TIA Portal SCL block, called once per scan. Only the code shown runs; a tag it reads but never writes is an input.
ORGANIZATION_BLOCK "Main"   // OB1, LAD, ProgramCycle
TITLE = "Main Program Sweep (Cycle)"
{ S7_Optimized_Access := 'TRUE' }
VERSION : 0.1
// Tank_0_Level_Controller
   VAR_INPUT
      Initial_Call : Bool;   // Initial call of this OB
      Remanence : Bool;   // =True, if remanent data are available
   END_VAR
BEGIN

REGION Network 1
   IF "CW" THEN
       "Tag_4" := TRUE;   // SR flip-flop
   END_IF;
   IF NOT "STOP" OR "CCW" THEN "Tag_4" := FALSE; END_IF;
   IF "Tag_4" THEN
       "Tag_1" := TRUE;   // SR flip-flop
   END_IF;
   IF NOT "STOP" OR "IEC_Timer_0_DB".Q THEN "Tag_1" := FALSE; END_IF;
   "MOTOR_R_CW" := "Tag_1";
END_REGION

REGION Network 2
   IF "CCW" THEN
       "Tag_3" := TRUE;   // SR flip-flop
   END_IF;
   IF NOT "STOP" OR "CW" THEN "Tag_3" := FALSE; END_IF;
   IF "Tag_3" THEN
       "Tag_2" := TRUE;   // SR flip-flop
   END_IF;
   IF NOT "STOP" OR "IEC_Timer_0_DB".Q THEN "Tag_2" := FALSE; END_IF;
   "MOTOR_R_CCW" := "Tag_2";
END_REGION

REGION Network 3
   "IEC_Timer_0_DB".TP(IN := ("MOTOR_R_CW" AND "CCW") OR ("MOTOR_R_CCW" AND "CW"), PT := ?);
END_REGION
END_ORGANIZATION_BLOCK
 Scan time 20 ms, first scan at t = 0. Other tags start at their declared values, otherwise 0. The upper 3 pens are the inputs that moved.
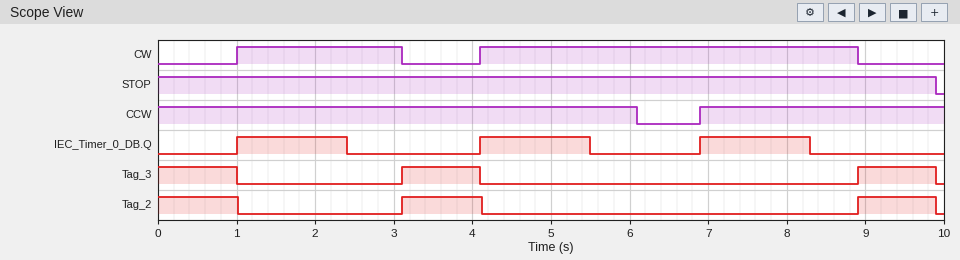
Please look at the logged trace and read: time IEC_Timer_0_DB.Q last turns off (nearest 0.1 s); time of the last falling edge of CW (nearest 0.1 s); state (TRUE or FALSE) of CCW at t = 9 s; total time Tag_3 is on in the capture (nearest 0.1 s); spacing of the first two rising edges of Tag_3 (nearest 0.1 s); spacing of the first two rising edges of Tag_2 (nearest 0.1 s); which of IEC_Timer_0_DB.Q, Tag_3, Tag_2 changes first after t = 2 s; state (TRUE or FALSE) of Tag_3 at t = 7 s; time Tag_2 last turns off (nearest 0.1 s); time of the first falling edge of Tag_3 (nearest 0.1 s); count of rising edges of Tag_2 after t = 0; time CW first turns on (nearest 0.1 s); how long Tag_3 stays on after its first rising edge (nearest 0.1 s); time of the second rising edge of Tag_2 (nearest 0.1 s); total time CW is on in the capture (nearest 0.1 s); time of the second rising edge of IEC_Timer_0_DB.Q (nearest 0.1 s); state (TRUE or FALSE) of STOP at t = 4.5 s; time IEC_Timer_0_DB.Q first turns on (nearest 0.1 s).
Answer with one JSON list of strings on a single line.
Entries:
["8.3 s", "8.9 s", "TRUE", "3.0 s", "5.8 s", "5.8 s", "IEC_Timer_0_DB.Q", "FALSE", "9.9 s", "1.0 s", "2", "1.0 s", "1.0 s", "8.9 s", "6.9 s", "4.1 s", "TRUE", "1.0 s"]
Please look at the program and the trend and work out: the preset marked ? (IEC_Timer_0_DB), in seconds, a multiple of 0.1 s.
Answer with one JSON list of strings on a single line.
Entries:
["1.4 s"]
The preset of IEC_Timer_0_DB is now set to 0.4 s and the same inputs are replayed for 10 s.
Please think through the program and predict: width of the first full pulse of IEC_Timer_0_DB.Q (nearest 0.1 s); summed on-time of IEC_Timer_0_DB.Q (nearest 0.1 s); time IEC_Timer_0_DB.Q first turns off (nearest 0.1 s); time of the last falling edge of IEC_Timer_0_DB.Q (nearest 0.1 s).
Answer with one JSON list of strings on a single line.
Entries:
["0.4 s", "1.2 s", "1.4 s", "7.3 s"]
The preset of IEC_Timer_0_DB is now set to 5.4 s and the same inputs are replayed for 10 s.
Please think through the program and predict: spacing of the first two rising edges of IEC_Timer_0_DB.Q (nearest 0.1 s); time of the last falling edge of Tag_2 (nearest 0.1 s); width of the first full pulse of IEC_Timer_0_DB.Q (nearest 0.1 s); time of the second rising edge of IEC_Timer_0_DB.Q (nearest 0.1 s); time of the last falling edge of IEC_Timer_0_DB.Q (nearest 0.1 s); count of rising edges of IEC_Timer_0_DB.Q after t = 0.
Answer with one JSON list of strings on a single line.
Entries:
["5.9 s", "1.0 s", "5.4 s", "6.9 s", "6.4 s", "2"]
